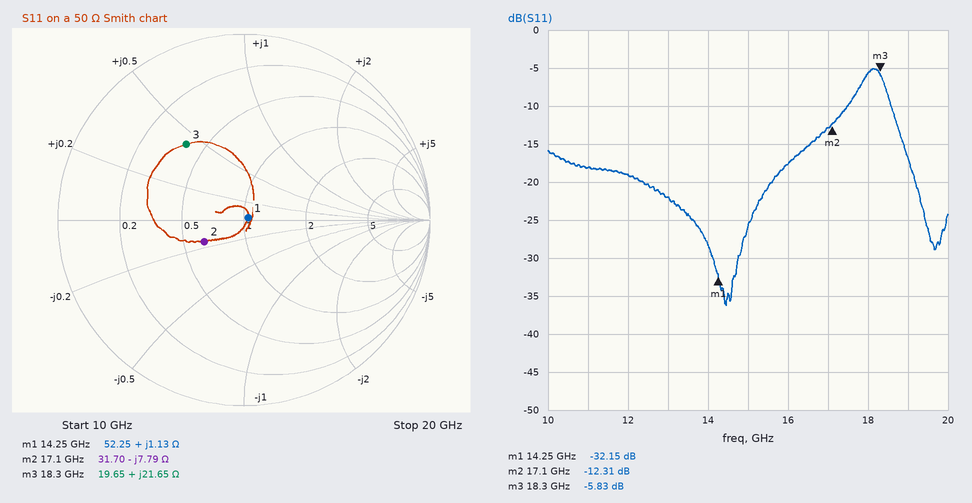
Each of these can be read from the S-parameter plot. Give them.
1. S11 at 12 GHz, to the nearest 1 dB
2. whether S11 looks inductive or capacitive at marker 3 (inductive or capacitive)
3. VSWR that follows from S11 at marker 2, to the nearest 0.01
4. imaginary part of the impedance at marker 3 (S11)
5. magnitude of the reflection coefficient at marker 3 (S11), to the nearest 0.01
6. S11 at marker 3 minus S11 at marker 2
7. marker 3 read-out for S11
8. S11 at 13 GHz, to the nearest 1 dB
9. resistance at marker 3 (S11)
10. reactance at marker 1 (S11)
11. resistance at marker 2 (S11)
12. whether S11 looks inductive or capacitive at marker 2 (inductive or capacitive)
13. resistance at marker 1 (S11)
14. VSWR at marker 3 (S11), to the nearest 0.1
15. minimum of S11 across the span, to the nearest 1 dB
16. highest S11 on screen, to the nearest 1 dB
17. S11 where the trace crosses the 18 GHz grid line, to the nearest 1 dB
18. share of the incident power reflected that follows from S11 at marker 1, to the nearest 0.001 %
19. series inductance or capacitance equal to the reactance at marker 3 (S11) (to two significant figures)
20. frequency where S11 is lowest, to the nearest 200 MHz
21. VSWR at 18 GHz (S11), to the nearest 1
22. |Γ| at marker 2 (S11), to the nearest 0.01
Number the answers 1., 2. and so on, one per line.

1. -19 dB
2. inductive
3. 1.64
4. +21.65 Ω
5. 0.51
6. 6.48 dB
7. -5.83 dB
8. -22 dB
9. 19.65 Ω
10. +1.13 Ω
11. 31.70 Ω
12. capacitive
13. 52.25 Ω
14. 3.1
15. -36 dB
16. -5 dB
17. -6 dB
18. 0.061 %
19. 190 pH
20. 14.4 GHz
21. 3
22. 0.24
